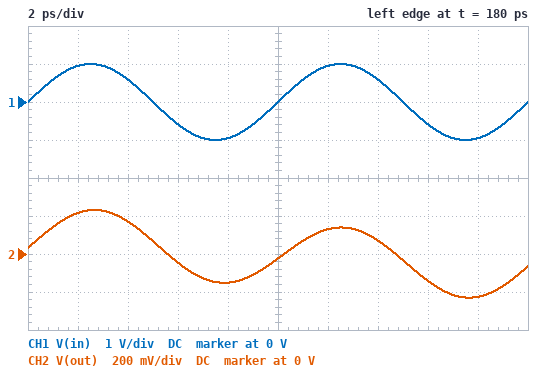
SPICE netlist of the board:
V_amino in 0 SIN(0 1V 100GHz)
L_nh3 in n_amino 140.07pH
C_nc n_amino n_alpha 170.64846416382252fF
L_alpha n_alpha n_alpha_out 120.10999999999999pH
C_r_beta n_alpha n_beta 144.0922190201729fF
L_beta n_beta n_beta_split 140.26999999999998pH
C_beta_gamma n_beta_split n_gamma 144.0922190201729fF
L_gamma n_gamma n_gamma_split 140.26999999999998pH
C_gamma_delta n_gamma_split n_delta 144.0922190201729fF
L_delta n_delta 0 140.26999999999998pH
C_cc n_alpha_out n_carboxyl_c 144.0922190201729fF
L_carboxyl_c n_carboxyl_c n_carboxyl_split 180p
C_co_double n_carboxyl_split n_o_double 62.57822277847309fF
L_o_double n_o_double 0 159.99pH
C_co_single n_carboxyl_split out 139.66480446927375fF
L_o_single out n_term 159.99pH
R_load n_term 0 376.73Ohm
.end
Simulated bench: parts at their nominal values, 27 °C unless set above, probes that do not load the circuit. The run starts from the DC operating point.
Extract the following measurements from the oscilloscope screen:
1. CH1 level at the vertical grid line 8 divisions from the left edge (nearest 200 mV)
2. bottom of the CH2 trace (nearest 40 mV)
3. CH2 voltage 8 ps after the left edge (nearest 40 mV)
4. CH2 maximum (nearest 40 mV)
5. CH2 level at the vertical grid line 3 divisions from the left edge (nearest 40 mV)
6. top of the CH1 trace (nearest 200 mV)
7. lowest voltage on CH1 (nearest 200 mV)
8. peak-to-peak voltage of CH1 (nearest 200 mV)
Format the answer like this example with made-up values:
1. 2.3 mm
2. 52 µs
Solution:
1. -600 mV
2. -240 mV
3. -160 mV
4. 240 mV
5. -40 mV
6. 1.0 V
7. -1.0 V
8. 2.0 V
